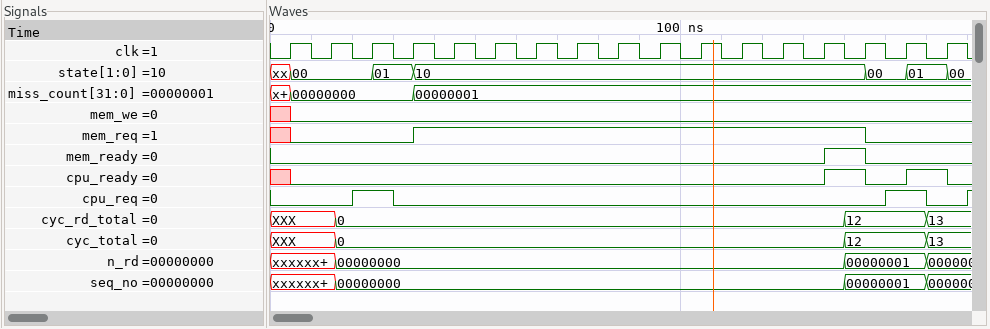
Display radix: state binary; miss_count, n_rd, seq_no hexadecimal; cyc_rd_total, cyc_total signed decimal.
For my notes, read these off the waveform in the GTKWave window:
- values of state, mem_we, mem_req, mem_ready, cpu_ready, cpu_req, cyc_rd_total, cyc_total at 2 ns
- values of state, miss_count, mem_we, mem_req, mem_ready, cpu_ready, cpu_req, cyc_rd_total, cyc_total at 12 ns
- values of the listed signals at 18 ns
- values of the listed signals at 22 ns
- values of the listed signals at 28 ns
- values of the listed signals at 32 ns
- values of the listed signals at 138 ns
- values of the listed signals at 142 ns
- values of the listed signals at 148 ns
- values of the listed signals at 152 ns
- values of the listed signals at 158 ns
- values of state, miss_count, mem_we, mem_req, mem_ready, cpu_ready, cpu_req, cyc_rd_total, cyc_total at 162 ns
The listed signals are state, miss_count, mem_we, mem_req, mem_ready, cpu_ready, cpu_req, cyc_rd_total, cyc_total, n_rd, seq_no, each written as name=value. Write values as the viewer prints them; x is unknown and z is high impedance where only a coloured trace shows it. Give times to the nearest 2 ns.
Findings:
state=xx, mem_we=x, mem_req=x, mem_ready=0, cpu_ready=x, cpu_req=0, cyc_rd_total=XXX, cyc_total=XXX
state=00, miss_count=00000000, mem_we=0, mem_req=0, mem_ready=0, cpu_ready=0, cpu_req=0, cyc_rd_total=XXX, cyc_total=XXX
state=00, miss_count=00000000, mem_we=0, mem_req=0, mem_ready=0, cpu_ready=0, cpu_req=0, cyc_rd_total=0, cyc_total=0, n_rd=00000000, seq_no=00000000
state=00, miss_count=00000000, mem_we=0, mem_req=0, mem_ready=0, cpu_ready=0, cpu_req=1, cyc_rd_total=0, cyc_total=0, n_rd=00000000, seq_no=00000000
state=01, miss_count=00000000, mem_we=0, mem_req=0, mem_ready=0, cpu_ready=0, cpu_req=1, cyc_rd_total=0, cyc_total=0, n_rd=00000000, seq_no=00000000
state=01, miss_count=00000000, mem_we=0, mem_req=0, mem_ready=0, cpu_ready=0, cpu_req=0, cyc_rd_total=0, cyc_total=0, n_rd=00000000, seq_no=00000000
state=10, miss_count=00000001, mem_we=0, mem_req=1, mem_ready=1, cpu_ready=1, cpu_req=0, cyc_rd_total=0, cyc_total=0, n_rd=00000000, seq_no=00000000
state=10, miss_count=00000001, mem_we=0, mem_req=1, mem_ready=1, cpu_ready=1, cpu_req=0, cyc_rd_total=12, cyc_total=12, n_rd=00000001, seq_no=00000001
state=00, miss_count=00000001, mem_we=0, mem_req=0, mem_ready=0, cpu_ready=0, cpu_req=0, cyc_rd_total=12, cyc_total=12, n_rd=00000001, seq_no=00000001
state=00, miss_count=00000001, mem_we=0, mem_req=0, mem_ready=0, cpu_ready=0, cpu_req=1, cyc_rd_total=12, cyc_total=12, n_rd=00000001, seq_no=00000001
state=01, miss_count=00000001, mem_we=0, mem_req=0, mem_ready=0, cpu_ready=1, cpu_req=1, cyc_rd_total=12, cyc_total=12, n_rd=00000001, seq_no=00000001
state=01, miss_count=00000001, mem_we=0, mem_req=0, mem_ready=0, cpu_ready=1, cpu_req=0, cyc_rd_total=13, cyc_total=13
